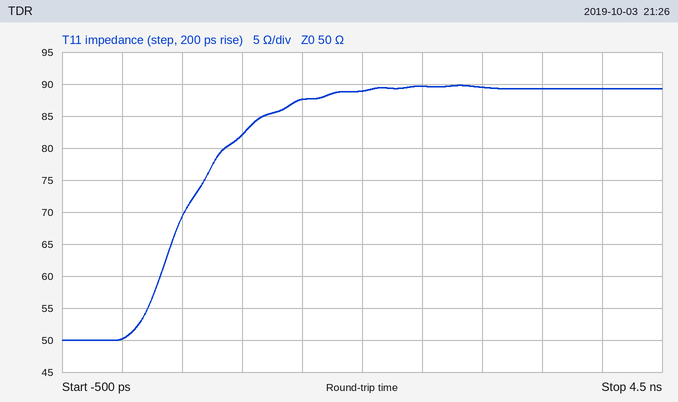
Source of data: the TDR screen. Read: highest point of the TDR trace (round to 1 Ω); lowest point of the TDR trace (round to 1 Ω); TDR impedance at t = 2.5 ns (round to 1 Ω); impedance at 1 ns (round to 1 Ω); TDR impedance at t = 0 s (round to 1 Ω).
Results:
90 Ω
50 Ω
90 Ω
82 Ω
50 Ω
